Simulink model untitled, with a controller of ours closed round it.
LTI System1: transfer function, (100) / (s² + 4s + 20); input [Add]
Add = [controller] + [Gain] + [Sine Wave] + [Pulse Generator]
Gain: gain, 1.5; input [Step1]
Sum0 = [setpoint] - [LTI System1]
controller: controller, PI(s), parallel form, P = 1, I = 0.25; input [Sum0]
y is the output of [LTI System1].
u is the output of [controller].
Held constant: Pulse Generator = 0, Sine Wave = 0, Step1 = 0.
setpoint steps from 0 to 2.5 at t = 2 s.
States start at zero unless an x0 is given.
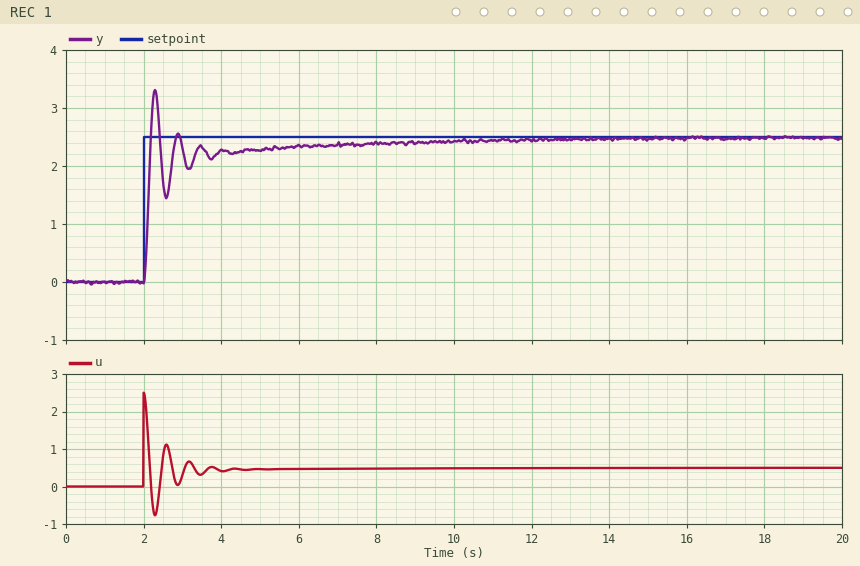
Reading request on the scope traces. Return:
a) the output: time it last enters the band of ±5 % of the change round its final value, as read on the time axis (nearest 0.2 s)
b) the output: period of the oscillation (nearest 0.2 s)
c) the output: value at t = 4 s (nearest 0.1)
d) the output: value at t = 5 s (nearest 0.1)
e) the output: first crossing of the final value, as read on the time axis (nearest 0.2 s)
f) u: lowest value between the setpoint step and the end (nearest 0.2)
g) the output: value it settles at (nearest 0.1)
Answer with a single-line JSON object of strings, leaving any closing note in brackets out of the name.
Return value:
{"the output: time it last enters the band of ±5 % of the change round its final value, as read on the time axis": "7.6 s", "the output: period of the oscillation": "0.6 s", "the output: value at t = 4 s": "2.3", "the output: value at t = 5 s": "2.3", "the output: first crossing of the final value, as read on the time axis": "2.2 s", "u: lowest value between the setpoint step and the end": "-0.8", "the output: value it settles at": "2.5"}
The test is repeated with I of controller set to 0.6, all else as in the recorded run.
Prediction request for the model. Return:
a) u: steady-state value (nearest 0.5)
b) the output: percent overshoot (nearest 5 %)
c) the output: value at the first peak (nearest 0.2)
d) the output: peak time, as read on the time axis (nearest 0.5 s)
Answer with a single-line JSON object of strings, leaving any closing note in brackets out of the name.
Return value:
{"u: steady-state value": "0.5", "the output: percent overshoot": "35 %", "the output: value at the first peak": "3.4", "the output: peak time, as read on the time axis": "2.5 s"}
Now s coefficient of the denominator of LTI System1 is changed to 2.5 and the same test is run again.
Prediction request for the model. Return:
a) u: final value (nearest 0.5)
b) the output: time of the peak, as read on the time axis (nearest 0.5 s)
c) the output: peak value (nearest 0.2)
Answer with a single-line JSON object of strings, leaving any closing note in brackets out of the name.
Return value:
{"u: final value": "0.5", "the output: time of the peak, as read on the time axis": "2.5 s", "the output: peak value": "3.6"}
